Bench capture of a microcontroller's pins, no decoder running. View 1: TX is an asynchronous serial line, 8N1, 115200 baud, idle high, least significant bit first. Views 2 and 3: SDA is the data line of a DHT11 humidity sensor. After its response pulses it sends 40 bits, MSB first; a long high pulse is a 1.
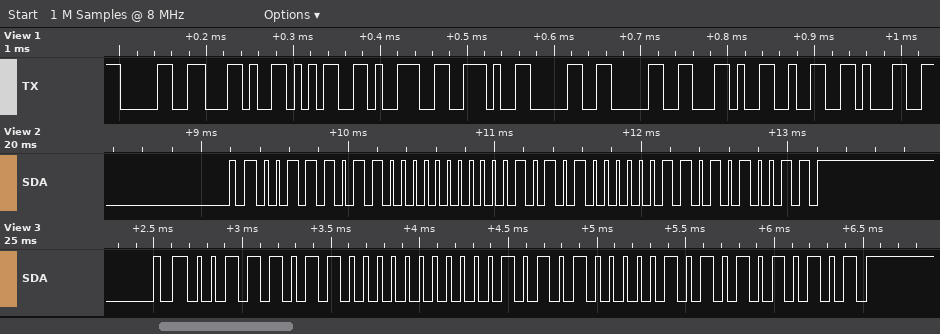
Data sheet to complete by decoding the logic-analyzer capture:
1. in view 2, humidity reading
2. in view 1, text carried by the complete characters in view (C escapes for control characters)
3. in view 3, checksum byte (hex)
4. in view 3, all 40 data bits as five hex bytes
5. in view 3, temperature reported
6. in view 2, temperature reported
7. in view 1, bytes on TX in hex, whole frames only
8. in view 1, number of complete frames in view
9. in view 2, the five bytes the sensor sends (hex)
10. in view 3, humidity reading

59 %
"0,59.00,21"
0x55
3B 00 15 05 55
21.5 °C
21.3 °C
0x30 0x2C 0x35 0x39 0x2E 0x30 0x30 0x2C 0x32 0x31
10
3B 00 15 03 53
59 %
